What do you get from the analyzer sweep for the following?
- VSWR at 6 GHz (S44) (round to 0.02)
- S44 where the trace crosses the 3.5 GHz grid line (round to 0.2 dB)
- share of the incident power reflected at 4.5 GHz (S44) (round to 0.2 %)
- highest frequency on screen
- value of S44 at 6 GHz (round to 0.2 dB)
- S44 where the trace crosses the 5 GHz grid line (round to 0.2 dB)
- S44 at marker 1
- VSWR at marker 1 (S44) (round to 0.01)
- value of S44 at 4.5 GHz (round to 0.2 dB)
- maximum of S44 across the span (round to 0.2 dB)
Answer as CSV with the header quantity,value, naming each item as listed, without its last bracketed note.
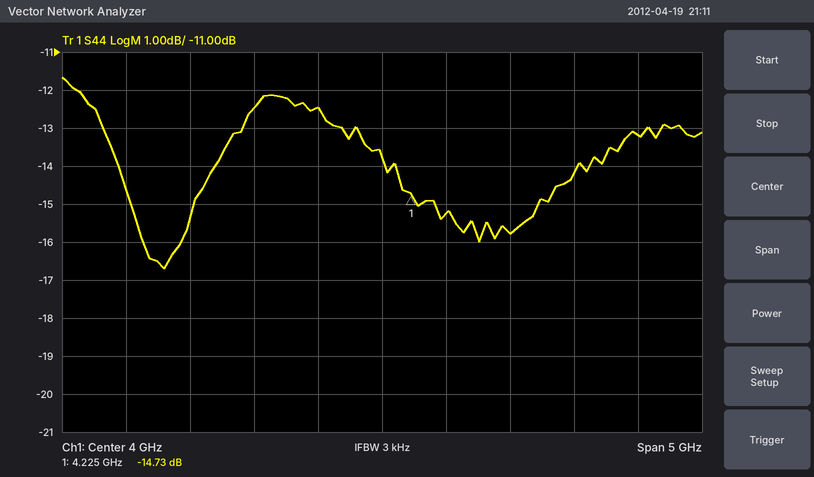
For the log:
quantity,value
VSWR at 6 GHz (S44),1.56
S44 where the trace crosses the 3.5 GHz grid line,-12.4 dB
share of the incident power reflected at 4.5 GHz (S44),3.0 %
highest frequency on screen,6.5 GHz
value of S44 at 6 GHz,-13.2 dB
S44 where the trace crosses the 5 GHz grid line,-15.8 dB
S44 at marker 1,-14.73 dB
VSWR at marker 1 (S44),1.45
value of S44 at 4.5 GHz,-15.2 dB
maximum of S44 across the span,-11.6 dB
